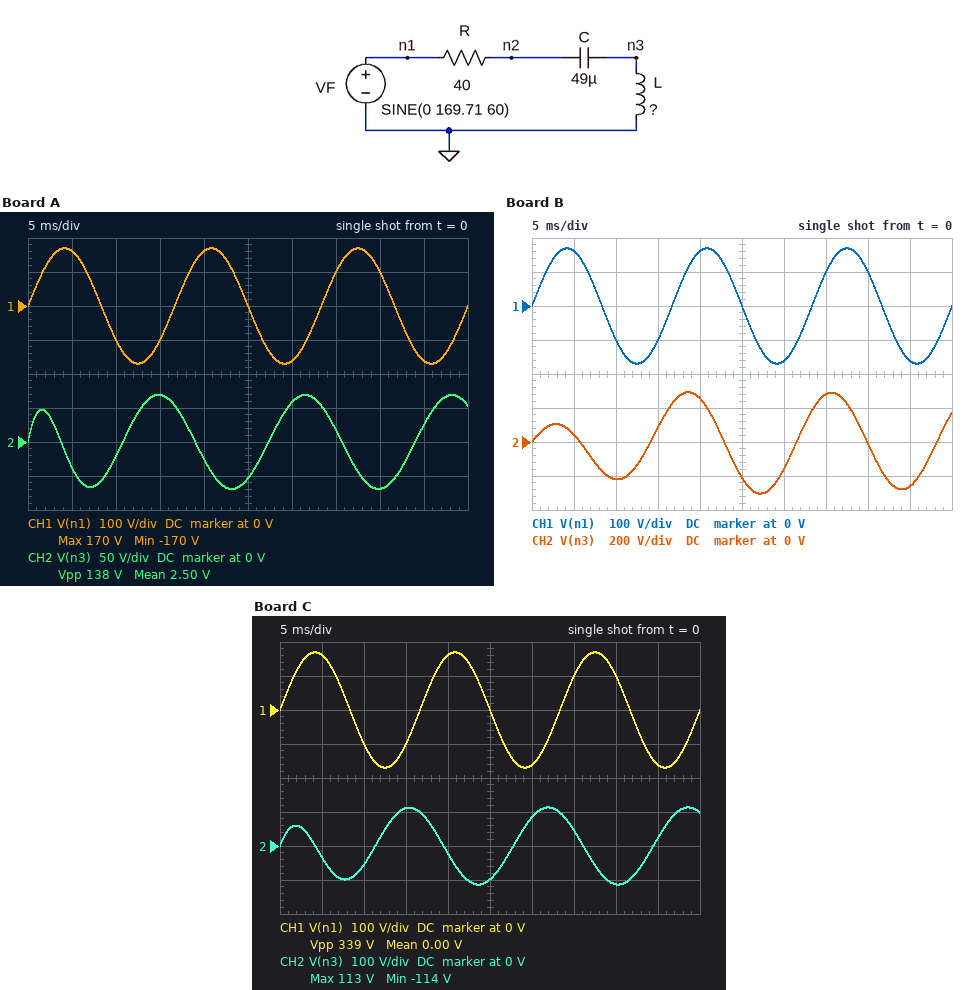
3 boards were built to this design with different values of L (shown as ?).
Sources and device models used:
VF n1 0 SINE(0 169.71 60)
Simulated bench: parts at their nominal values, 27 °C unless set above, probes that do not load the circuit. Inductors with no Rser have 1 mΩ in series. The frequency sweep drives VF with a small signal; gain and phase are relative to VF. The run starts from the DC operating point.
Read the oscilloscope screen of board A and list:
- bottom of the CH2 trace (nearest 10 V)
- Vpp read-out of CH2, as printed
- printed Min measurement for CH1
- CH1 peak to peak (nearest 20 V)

-70 V
138 V
-170 V
340 V
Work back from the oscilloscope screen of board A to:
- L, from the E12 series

56 mH
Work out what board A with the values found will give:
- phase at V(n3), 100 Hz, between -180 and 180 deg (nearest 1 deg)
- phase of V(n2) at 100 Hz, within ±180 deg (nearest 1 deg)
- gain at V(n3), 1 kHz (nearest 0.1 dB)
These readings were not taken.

86 deg
86 deg
0 dB
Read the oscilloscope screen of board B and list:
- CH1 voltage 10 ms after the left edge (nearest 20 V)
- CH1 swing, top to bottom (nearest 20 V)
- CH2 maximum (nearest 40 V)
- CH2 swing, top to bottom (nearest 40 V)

-100 V
340 V
280 V
600 V
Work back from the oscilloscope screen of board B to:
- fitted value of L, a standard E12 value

270 mH
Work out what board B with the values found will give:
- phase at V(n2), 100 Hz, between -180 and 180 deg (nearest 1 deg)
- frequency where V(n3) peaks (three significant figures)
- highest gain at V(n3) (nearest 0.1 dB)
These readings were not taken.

16 deg
47.3 Hz
5.7 dB
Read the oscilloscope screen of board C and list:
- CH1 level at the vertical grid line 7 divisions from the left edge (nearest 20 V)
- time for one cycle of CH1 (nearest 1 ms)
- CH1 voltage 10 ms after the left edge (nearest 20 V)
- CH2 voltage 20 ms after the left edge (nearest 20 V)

100 V
17 ms
-100 V
-20 V
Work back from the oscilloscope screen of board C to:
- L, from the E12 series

82 mH
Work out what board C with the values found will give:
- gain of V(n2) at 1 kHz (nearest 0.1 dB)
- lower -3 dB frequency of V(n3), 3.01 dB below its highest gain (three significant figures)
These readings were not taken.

0 dB
67.7 Hz
